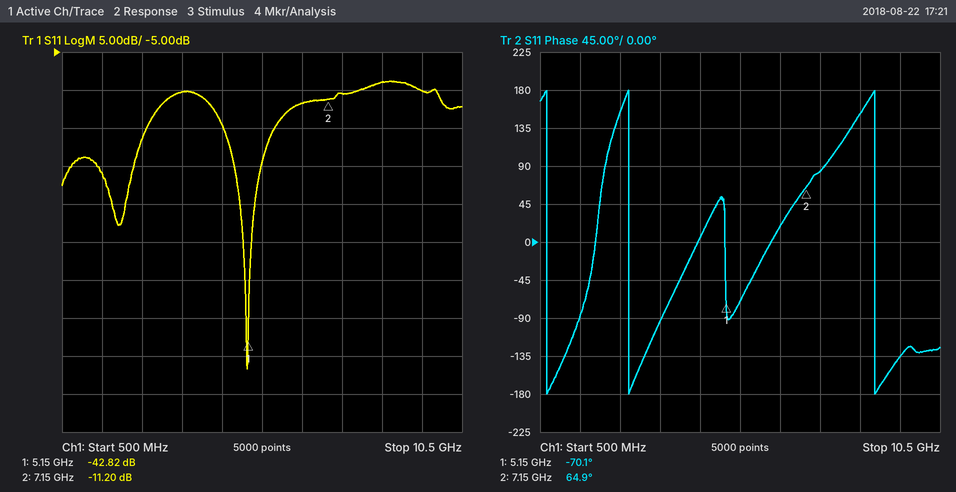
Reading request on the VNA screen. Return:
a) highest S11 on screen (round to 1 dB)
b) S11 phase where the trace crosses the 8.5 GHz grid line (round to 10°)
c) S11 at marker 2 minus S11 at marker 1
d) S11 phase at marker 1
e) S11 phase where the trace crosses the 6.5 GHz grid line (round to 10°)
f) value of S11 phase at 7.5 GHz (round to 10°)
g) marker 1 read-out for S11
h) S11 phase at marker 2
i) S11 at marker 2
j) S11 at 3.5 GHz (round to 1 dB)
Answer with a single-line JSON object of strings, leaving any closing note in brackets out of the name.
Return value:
{"highest S11 on screen": "-9 dB", "S11 phase where the trace crosses the 8.5 GHz grid line": "150°", "S11 at marker 2 minus S11 at marker 1": "31.62 dB", "S11 phase at marker 1": "-70.1°", "S11 phase where the trace crosses the 6.5 GHz grid line": "20°", "value of S11 phase at 7.5 GHz": "80°", "marker 1 read-out for S11": "-42.82 dB", "S11 phase at marker 2": "64.9°", "S11 at marker 2": "-11.20 dB", "S11 at 3.5 GHz": "-10 dB"}
